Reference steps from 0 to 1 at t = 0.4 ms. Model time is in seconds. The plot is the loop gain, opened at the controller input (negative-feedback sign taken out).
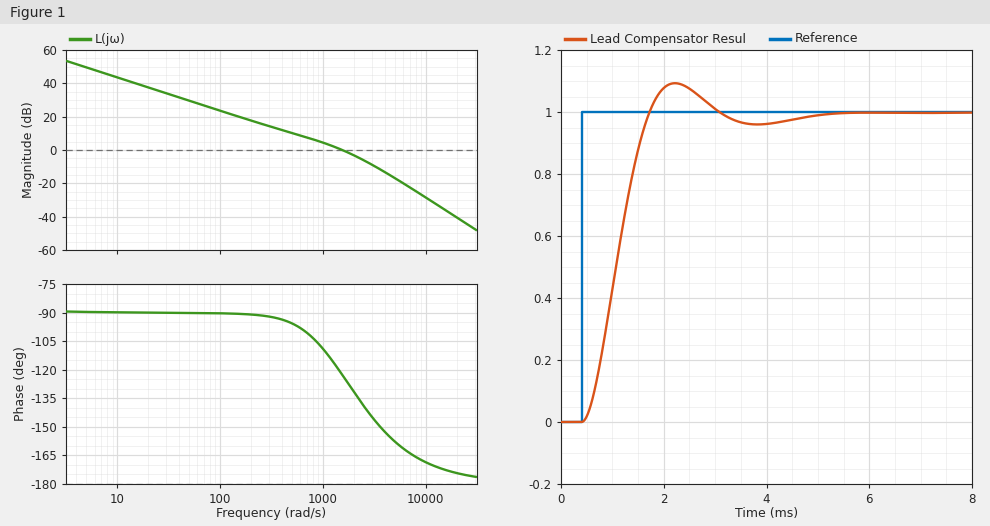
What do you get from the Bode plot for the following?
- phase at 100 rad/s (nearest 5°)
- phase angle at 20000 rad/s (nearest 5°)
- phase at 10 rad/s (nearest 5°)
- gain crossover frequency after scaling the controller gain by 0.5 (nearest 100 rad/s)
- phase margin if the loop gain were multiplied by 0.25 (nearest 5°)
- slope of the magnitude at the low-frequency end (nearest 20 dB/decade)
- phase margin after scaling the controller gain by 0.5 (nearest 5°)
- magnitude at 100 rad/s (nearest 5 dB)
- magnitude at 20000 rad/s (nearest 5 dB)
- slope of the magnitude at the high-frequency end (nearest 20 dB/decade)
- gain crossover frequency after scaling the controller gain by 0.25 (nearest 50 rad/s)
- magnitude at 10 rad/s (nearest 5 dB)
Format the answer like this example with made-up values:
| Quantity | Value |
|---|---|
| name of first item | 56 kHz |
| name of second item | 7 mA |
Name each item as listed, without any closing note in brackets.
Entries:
| Quantity | Value |
|---|---|
| phase at 100 rad/s | -90° |
| phase angle at 20000 rad/s | -175° |
| phase at 10 rad/s | -90° |
| gain crossover frequency after scaling the controller gain by 0.5 | 800 rad/s |
| phase margin if the loop gain were multiplied by 0.25 | 85° |
| slope of the magnitude at the low-frequency end | -20 dB/decade |
| phase margin after scaling the controller gain by 0.5 | 75° |
| magnitude at 100 rad/s | 25 dB |
| magnitude at 20000 rad/s | -40 dB |
| slope of the magnitude at the high-frequency end | -40 dB/decade |
| gain crossover frequency after scaling the controller gain by 0.25 | 400 rad/s |
| magnitude at 10 rad/s | 45 dB |
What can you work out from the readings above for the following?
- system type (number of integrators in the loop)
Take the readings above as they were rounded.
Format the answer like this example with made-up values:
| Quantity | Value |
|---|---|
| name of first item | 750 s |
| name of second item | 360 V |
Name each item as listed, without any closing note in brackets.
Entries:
| Quantity | Value |
|---|---|
| system type | 1 |
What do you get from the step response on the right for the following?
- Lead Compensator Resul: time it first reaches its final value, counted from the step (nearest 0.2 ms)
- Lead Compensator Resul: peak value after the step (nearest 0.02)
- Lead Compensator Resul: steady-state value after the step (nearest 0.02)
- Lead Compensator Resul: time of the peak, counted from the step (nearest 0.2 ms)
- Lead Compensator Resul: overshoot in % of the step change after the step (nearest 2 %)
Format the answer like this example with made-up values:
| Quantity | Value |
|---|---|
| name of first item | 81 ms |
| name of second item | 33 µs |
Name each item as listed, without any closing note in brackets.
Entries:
| Quantity | Value |
|---|---|
| Lead Compensator Resul: time it first reaches its final value, counted from the step | 1.4 ms |
| Lead Compensator Resul: peak value after the step | 1.10 |
| Lead Compensator Resul: steady-state value after the step | 1.00 |
| Lead Compensator Resul: time of the peak, counted from the step | 1.8 ms |
| Lead Compensator Resul: overshoot in % of the step change after the step | 10 % |
